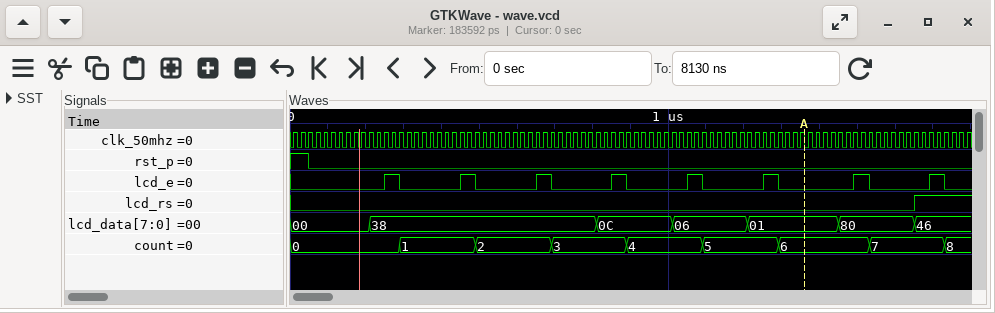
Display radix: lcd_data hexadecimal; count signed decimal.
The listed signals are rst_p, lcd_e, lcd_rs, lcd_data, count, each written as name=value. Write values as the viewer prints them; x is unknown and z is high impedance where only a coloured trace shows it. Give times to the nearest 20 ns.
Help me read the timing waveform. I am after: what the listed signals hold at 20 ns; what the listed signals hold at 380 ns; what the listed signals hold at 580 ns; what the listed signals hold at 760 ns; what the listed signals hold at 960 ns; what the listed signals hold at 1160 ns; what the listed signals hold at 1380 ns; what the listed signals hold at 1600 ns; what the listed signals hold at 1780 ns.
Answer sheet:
rst_p=1, lcd_e=0, lcd_rs=0, lcd_data=00, count=0
rst_p=0, lcd_e=0, lcd_rs=0, lcd_data=38, count=1
rst_p=0, lcd_e=0, lcd_rs=0, lcd_data=38, count=2
rst_p=0, lcd_e=0, lcd_rs=0, lcd_data=38, count=3
rst_p=0, lcd_e=0, lcd_rs=0, lcd_data=0C, count=4
rst_p=0, lcd_e=0, lcd_rs=0, lcd_data=06, count=5
rst_p=0, lcd_e=0, lcd_rs=0, lcd_data=01, count=6
rst_p=0, lcd_e=0, lcd_rs=0, lcd_data=80, count=7
rst_p=0, lcd_e=0, lcd_rs=1, lcd_data=46, count=8
